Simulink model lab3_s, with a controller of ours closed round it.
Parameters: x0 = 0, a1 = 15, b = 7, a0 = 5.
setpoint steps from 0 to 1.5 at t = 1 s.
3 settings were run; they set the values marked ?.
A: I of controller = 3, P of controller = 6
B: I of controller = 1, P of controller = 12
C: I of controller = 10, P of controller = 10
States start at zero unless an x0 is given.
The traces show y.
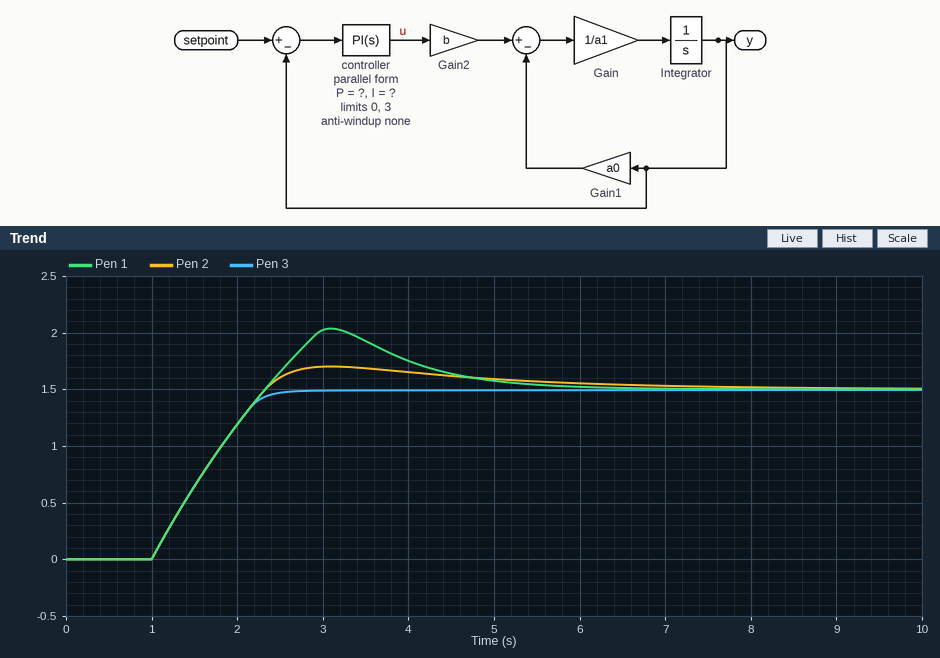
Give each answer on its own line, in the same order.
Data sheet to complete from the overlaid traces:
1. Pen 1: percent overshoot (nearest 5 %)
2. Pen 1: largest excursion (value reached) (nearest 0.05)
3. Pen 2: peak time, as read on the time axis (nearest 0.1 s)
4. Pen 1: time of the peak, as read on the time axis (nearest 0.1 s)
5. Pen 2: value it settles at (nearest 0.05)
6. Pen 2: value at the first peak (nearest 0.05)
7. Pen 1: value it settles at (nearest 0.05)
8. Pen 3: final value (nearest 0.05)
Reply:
35 %
2.05
3.1 s
3.1 s
1.50
1.70
1.50
1.50
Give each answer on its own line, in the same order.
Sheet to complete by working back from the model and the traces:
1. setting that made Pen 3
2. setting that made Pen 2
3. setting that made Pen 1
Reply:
B
A
C
